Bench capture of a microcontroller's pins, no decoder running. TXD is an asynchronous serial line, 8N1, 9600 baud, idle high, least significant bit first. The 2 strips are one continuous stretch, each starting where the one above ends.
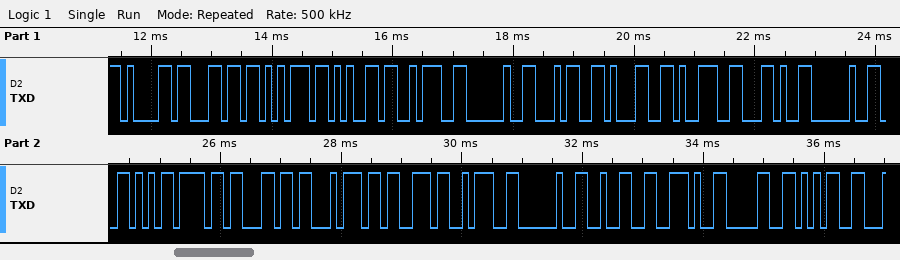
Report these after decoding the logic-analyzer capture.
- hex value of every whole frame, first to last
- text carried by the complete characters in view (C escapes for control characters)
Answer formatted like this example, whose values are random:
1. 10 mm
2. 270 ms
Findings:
1. 61 6C 75 65 3A 20 34 31 39 2C 20 56 6F 6C 74 73 3A 20 32 2E 30 35
2. "alue: 419, Volts: 2.05"
